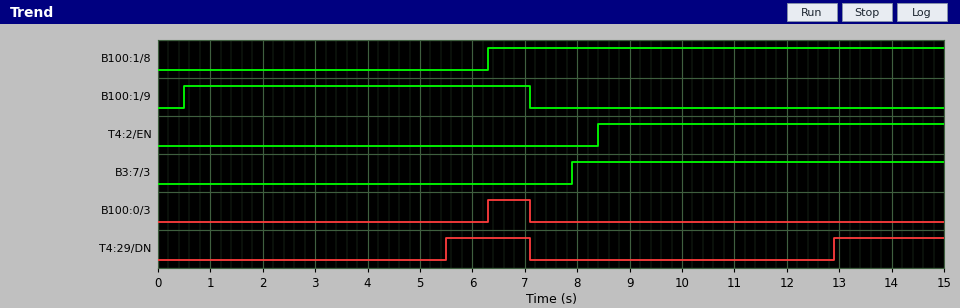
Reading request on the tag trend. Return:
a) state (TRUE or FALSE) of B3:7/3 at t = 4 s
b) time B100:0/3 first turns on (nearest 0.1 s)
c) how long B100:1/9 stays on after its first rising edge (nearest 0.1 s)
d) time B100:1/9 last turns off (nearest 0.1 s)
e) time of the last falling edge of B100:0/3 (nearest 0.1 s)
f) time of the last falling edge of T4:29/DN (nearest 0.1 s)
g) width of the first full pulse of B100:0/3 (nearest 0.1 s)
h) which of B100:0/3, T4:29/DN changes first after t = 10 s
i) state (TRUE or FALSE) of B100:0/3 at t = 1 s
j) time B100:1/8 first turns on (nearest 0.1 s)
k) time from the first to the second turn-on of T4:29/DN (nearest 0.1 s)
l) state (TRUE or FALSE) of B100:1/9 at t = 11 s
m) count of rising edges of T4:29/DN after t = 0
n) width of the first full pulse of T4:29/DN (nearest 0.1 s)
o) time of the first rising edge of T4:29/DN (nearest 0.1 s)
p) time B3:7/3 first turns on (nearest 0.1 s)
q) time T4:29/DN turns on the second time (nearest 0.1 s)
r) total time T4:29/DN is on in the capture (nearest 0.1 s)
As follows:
FALSE
6.3 s
6.6 s
7.1 s
7.1 s
7.1 s
0.8 s
T4:29/DN
FALSE
6.3 s
7.4 s
FALSE
2
1.6 s
5.5 s
7.9 s
12.9 s
3.7 s
